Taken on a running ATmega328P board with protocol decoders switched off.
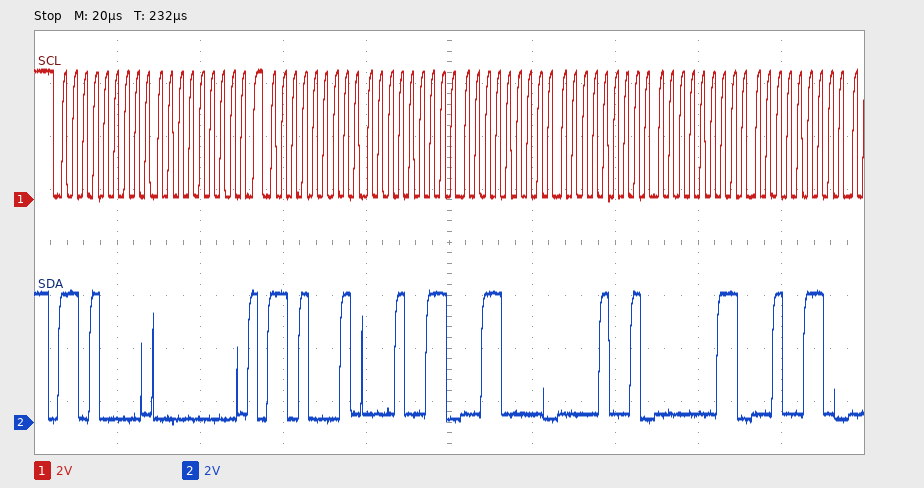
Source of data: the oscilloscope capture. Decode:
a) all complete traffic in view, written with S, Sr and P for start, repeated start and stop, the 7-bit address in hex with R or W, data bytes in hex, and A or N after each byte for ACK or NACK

S 68W A 00 A Sr 68R A 13 A 30 A 09 A 03 A 26 A
